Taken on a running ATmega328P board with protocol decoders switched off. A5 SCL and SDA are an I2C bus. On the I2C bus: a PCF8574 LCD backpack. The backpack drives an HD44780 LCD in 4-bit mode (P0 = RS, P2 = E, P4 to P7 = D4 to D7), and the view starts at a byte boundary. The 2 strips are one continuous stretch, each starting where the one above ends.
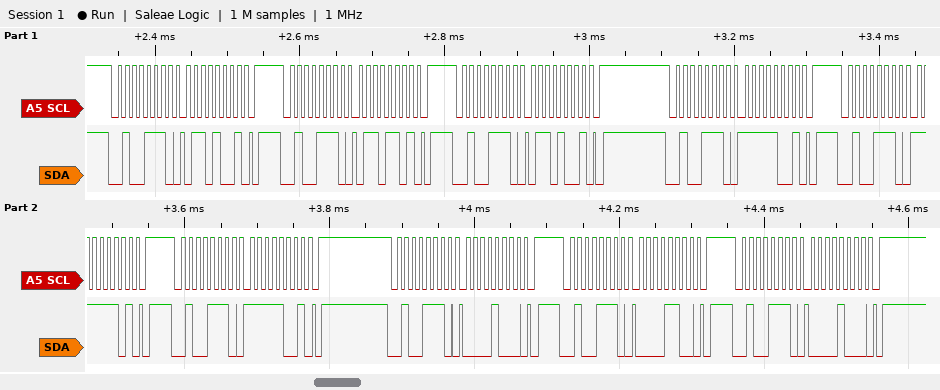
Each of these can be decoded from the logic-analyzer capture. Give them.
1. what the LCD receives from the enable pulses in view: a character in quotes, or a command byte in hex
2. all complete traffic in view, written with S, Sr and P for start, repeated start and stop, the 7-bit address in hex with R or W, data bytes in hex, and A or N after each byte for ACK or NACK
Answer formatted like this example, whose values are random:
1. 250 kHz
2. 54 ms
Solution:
1. 'o'
2. S 27W A 69 A P S 27W A 6D A P S 27W A 69 A P S 27W A F9 A P S 27W A FD A P S 27W A F9 A P S 27W A 08 A P S 27W A 0C A P S 27W A 08 A P
